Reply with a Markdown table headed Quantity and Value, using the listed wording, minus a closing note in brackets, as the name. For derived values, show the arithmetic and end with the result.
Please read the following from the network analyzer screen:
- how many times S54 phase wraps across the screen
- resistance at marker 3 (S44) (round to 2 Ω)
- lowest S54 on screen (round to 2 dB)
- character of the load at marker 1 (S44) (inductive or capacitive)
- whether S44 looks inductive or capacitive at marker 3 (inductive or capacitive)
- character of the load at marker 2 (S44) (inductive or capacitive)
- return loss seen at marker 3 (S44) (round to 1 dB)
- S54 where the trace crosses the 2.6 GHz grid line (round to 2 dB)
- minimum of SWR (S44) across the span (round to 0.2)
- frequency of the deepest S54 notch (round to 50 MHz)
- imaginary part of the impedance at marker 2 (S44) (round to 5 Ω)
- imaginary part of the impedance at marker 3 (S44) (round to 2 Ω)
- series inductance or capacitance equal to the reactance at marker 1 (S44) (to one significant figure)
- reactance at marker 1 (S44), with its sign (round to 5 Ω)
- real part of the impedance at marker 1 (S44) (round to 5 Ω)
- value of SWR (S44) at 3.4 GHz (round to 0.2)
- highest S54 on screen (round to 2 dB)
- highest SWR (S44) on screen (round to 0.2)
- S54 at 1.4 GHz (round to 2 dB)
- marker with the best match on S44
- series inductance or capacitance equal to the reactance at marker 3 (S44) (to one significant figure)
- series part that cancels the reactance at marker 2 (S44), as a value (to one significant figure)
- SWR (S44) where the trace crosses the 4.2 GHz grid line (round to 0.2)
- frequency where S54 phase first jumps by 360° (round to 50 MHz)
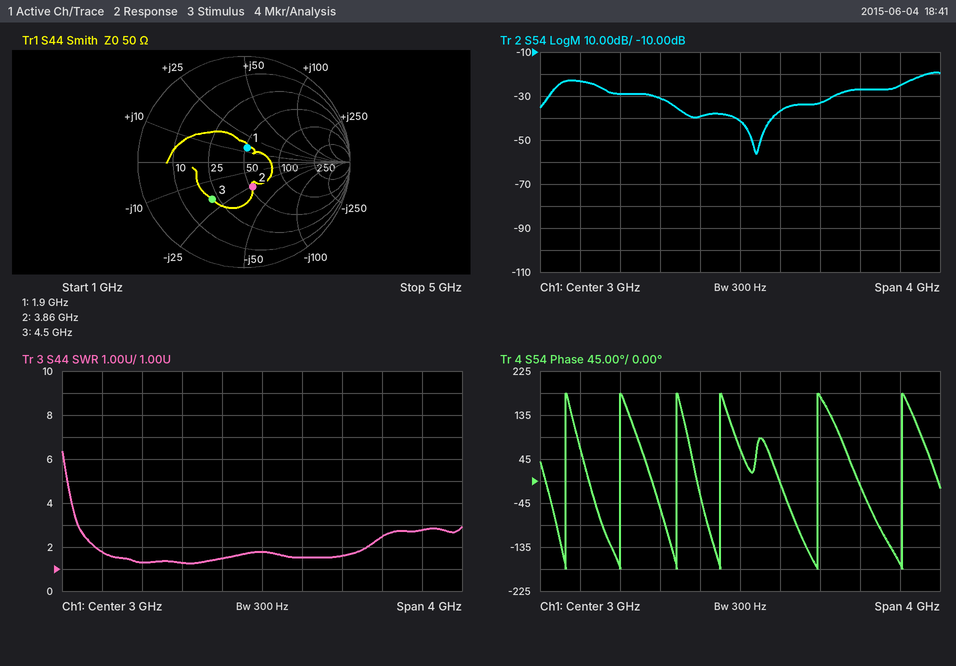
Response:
| Quantity | Value |
|---|---|
| how many times S54 phase wraps across the screen | 6 |
| resistance at marker 3 (S44) | 22 Ω |
| lowest S54 on screen | -56 dB |
| character of the load at marker 1 (S44) | inductive |
| whether S44 looks inductive or capacitive at marker 3 | capacitive |
| character of the load at marker 2 (S44) | capacitive |
| return loss seen at marker 3 (S44) | 7 dB |
| S54 where the trace crosses the 2.6 GHz grid line | -40 dB |
| minimum of SWR (S44) across the span | 1.2 |
| frequency of the deepest S54 notch | 3.15 GHz |
| imaginary part of the impedance at marker 2 (S44) | -25 Ω |
| imaginary part of the impedance at marker 3 (S44) | -20 Ω |
| series inductance or capacitance equal to the reactance at marker 1 (S44) | L = 15 Ω/(2π × 1.9 GHz) ≈ 1 nH |
| reactance at marker 1 (S44), with its sign | +15 Ω |
| real part of the impedance at marker 1 (S44) | 50 Ω |
| value of SWR (S44) at 3.4 GHz | 1.6 |
| highest S54 on screen | -20 dB |
| highest SWR (S44) on screen | 6.4 |
| S54 at 1.4 GHz | -24 dB |
| marker with the best match on S44 | marker 1 |
| series inductance or capacitance equal to the reactance at marker 3 (S44) | C = 1/(2π × 4.5 GHz × 20 Ω) ≈ 2 pF |
| series part that cancels the reactance at marker 2 (S44), as a value | L = 25 Ω/(2π × 3.86 GHz) ≈ 1 nH |
| SWR (S44) where the trace crosses the 4.2 GHz grid line | 2.4 |
| frequency where S54 phase first jumps by 360° | 1.25 GHz |
